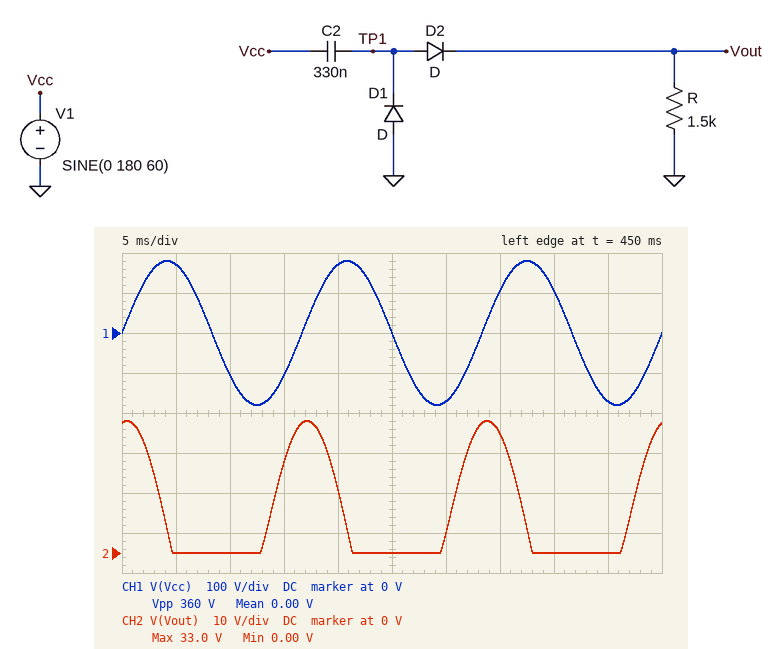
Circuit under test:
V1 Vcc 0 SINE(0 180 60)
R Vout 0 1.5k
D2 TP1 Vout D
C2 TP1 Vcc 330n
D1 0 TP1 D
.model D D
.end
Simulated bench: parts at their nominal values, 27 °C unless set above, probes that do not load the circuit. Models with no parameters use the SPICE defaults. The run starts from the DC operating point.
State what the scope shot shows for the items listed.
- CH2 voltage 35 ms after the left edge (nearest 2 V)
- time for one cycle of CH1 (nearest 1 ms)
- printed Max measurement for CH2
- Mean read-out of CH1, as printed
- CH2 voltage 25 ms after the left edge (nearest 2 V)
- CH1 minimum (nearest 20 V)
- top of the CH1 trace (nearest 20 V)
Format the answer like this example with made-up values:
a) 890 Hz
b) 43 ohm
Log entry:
a) 30 V
b) 17 ms
c) 33.0 V
d) 0.00 V
e) 0 V
f) -180 V
g) 180 V
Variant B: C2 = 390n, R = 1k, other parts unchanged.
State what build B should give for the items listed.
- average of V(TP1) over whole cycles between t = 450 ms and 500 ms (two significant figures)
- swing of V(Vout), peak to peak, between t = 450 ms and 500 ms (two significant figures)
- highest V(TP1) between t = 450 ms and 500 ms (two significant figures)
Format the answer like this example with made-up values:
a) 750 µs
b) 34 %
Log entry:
a) 8.4 V
b) 26 V
c) 27 V
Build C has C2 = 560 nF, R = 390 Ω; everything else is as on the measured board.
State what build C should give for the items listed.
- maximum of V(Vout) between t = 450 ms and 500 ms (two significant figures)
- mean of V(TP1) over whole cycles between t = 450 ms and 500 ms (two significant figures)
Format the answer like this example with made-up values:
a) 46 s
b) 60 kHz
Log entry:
a) 15 V
b) 4.7 V
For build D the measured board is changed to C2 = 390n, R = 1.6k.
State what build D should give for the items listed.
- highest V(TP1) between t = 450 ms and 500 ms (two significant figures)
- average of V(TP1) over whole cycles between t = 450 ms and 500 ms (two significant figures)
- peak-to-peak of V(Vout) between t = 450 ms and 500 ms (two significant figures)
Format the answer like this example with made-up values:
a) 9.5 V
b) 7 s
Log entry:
a) 42 V
b) 13 V
c) 41 V
